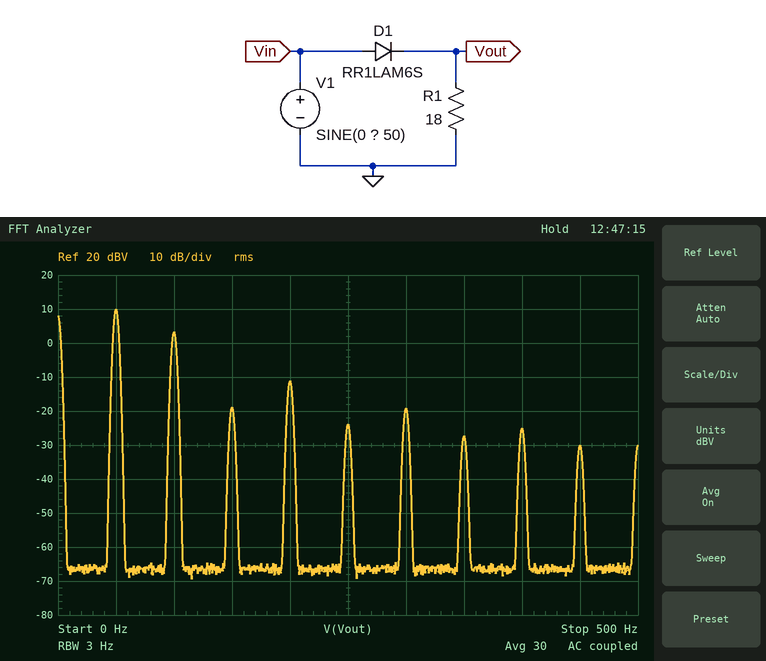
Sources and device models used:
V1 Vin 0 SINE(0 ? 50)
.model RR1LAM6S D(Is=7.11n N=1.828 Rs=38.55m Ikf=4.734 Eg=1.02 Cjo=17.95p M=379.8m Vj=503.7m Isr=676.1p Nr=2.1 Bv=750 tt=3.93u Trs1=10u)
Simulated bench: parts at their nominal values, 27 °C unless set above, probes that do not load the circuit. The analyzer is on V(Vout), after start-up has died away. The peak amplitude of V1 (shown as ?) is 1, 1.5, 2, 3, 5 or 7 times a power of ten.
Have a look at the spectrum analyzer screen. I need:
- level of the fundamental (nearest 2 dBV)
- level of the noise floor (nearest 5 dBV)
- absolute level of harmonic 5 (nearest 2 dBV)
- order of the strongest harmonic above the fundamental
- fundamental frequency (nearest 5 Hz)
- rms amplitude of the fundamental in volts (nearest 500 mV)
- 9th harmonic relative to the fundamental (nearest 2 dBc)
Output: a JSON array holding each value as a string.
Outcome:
["10 dBV", "-65 dBV", "-24 dBV", "2", "50 Hz", "3.0 V", "-40 dBc"]
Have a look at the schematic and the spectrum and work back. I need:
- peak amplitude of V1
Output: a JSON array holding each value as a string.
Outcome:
["10 V"]
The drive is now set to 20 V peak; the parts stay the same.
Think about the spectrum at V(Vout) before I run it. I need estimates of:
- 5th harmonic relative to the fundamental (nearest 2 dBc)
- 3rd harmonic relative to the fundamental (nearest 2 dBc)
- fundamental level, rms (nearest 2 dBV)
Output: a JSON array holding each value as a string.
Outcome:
["-40 dBc", "-34 dBc", "16 dBV"]
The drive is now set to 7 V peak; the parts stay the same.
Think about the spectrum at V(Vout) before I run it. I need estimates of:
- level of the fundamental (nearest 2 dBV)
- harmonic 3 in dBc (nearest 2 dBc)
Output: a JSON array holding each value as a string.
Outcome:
["6 dBV", "-26 dBc"]
